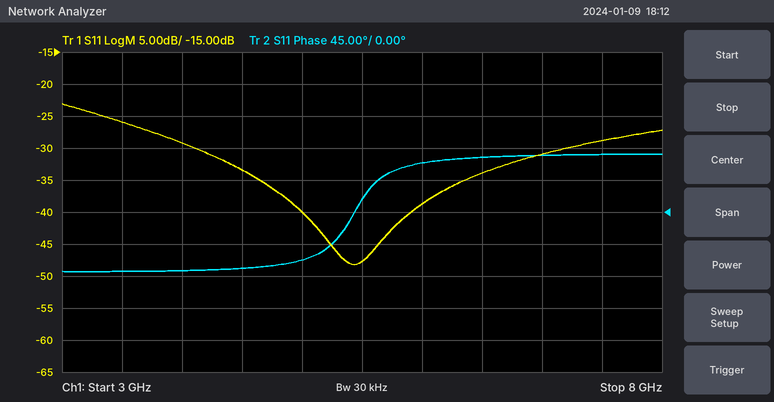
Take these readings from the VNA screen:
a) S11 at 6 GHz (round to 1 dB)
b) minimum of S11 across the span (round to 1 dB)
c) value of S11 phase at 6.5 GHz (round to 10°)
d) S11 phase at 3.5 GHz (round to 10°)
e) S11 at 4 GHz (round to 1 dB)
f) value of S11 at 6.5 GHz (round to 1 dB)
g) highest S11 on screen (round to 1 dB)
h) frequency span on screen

-39 dB
-48 dB
80°
-80°
-29 dB
-34 dB
-23 dB
5 GHz
